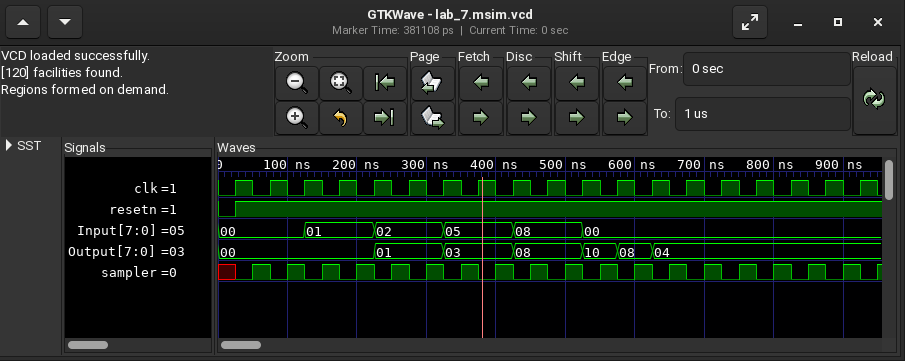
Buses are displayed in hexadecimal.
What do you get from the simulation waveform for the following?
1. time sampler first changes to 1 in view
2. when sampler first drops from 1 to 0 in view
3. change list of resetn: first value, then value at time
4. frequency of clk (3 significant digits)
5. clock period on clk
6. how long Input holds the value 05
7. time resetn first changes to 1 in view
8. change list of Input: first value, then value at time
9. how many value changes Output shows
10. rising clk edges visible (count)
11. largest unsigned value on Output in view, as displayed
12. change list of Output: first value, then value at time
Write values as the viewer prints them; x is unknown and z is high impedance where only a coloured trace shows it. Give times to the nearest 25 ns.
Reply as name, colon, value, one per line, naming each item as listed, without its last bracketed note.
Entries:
time sampler first changes to 1 in view: 50 ns
when sampler first drops from 1 to 0 in view: 75 ns
change list of resetn: first value, then value at time: 0, 1 at 25 ns
frequency of clk: 20.0 MHz
clock period on clk: 50 ns
how long Input holds the value 05: 100 ns
time resetn first changes to 1 in view: 25 ns
change list of Input: first value, then value at time: 00, 01 at 125 ns, 02 at 225 ns, 05 at 325 ns, 08 at 425 ns, 00 at 525 ns
how many value changes Output shows: 6
rising clk edges visible: 19
largest unsigned value on Output in view, as displayed: 10
change list of Output: first value, then value at time: 00, 01 at 225 ns, 03 at 325 ns, 08 at 425 ns, 10 at 525 ns, 08 at 575 ns, 04 at 625 ns
